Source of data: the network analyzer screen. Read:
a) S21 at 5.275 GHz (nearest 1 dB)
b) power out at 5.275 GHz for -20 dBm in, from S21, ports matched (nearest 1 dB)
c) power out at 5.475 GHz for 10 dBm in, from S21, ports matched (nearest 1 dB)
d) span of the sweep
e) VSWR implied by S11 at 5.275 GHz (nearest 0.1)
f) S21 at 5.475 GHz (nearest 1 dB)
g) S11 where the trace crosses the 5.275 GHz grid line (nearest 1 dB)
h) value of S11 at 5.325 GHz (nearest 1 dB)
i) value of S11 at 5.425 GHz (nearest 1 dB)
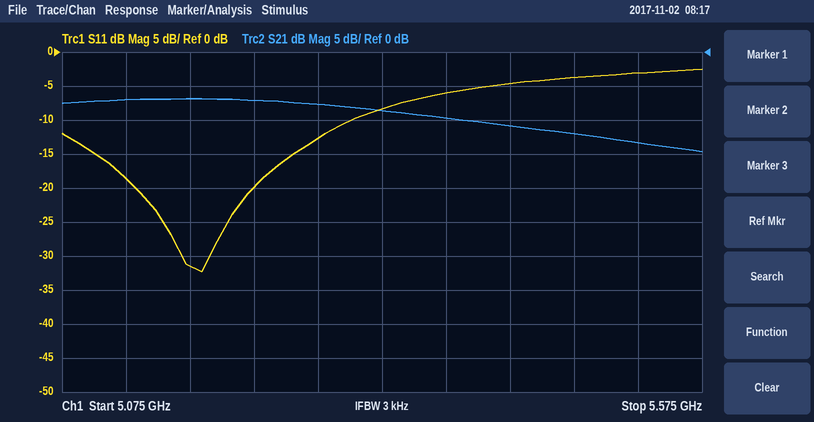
-8 dB
-28 dBm
-2 dBm
500 MHz
1.6
-12 dB
-13 dB
-8 dB
-5 dB
